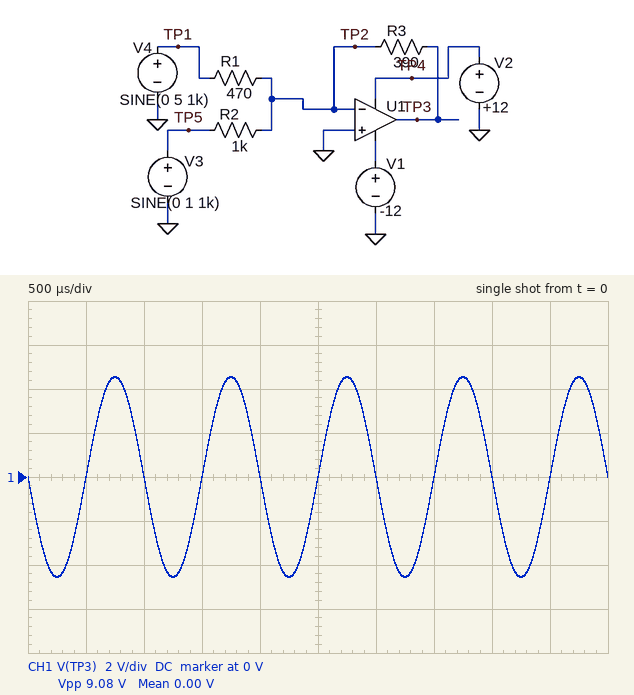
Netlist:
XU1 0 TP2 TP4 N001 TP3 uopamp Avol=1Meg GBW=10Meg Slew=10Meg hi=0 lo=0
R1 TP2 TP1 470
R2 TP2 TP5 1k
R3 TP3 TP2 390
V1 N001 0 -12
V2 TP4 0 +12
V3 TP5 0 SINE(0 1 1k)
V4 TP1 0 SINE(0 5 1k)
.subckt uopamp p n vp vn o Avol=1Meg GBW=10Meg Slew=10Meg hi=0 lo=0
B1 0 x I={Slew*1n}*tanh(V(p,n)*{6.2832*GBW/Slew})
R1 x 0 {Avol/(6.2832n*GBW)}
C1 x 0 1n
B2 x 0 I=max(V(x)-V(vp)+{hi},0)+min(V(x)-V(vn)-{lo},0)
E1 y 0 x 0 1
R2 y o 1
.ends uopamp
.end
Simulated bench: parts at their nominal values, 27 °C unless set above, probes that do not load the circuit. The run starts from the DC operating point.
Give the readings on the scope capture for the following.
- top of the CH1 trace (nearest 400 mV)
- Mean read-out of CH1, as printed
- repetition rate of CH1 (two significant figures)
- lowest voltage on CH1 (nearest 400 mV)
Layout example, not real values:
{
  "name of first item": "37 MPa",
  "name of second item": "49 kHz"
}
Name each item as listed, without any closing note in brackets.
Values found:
{
  "top of the CH1 trace": "4.4 V",
  "Mean read-out of CH1, as printed": "0.00 V",
  "repetition rate of CH1": "1.0 kHz",
  "lowest voltage on CH1": "-4.4 V"
}
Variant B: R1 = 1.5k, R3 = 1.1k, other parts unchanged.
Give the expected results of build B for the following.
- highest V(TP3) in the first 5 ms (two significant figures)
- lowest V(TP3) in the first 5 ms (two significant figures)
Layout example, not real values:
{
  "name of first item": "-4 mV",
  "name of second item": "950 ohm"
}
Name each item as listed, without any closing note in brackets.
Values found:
{
  "highest V(TP3) in the first 5 ms": "4.8 V",
  "lowest V(TP3) in the first 5 ms": "-4.8 V"
}
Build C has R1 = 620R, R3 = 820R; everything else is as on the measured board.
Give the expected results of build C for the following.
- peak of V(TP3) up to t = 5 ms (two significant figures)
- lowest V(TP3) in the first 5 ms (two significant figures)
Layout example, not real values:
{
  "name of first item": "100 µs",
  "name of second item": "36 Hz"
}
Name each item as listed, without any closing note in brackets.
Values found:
{
  "peak of V(TP3) up to t = 5 ms": "7.4 V",
  "lowest V(TP3) in the first 5 ms": "-7.4 V"
}
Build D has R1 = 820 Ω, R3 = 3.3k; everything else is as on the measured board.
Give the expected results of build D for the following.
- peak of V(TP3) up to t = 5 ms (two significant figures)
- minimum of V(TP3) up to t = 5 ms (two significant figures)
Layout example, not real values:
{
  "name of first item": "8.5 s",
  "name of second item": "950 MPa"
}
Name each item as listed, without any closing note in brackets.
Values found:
{
  "peak of V(TP3) up to t = 5 ms": "12 V",
  "minimum of V(TP3) up to t = 5 ms": "-12 V"
}
